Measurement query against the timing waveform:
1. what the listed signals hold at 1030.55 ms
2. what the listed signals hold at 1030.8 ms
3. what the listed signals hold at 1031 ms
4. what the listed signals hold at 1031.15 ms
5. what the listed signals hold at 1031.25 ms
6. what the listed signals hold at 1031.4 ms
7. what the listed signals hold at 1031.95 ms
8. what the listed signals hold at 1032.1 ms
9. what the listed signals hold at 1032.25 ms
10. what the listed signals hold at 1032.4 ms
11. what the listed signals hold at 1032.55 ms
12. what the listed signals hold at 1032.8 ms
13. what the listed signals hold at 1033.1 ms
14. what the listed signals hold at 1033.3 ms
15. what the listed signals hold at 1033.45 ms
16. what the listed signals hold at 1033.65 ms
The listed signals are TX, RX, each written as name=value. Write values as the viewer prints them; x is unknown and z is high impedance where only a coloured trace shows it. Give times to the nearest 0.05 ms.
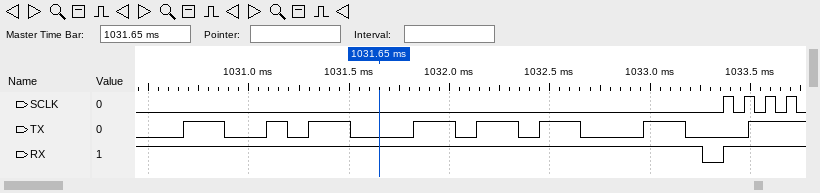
TX=0, RX=1
TX=1, RX=1
TX=0, RX=1
TX=1, RX=1
TX=0, RX=1
TX=1, RX=1
TX=1, RX=1
TX=0, RX=1
TX=1, RX=1
TX=0, RX=1
TX=1, RX=1
TX=0, RX=1
TX=1, RX=1
TX=0, RX=0
TX=0, RX=1
TX=1, RX=1
